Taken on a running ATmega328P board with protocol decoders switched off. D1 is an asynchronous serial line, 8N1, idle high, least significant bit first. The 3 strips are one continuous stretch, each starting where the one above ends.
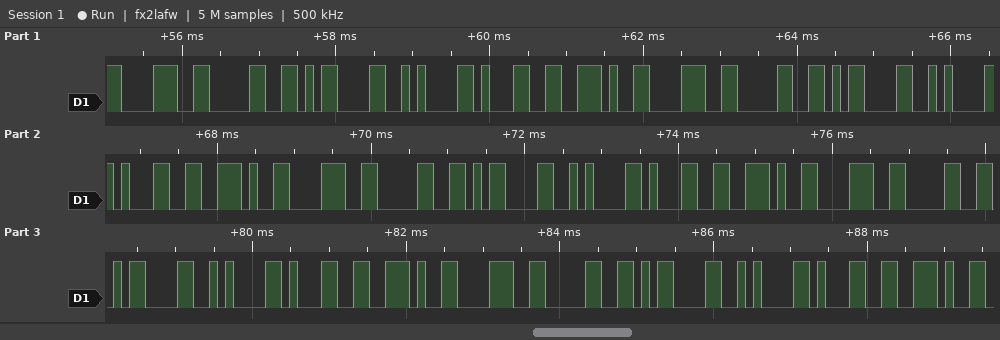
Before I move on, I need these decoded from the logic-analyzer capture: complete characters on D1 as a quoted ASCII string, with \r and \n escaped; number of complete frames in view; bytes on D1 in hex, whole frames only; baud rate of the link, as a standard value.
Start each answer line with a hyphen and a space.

- "80\r\n1.80\r\n1.80\r\n1.80\r\n1.80\r\n1."
- 30
- 38 30 0D 0A 31 2E 38 30 0D 0A 31 2E 38 30 0D 0A 31 2E 38 30 0D 0A 31 2E 38 30 0D 0A 31 2E
- 9600 baud
